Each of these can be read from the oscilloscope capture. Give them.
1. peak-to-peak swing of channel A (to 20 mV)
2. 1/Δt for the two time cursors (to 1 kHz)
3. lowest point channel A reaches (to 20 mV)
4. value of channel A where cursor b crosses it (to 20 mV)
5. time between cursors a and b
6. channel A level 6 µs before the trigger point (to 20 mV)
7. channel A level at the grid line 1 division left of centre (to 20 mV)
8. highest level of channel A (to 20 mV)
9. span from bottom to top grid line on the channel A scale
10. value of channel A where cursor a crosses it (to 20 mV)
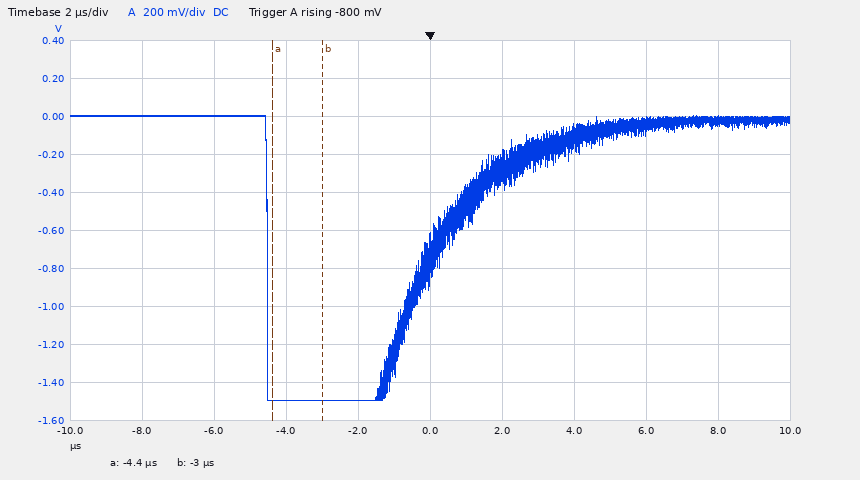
1.50 V
714 kHz
-1.50 V
-1.50 V
1.4 µs
0 mV
-1.50 V
0 mV
2 V
-1.50 V
